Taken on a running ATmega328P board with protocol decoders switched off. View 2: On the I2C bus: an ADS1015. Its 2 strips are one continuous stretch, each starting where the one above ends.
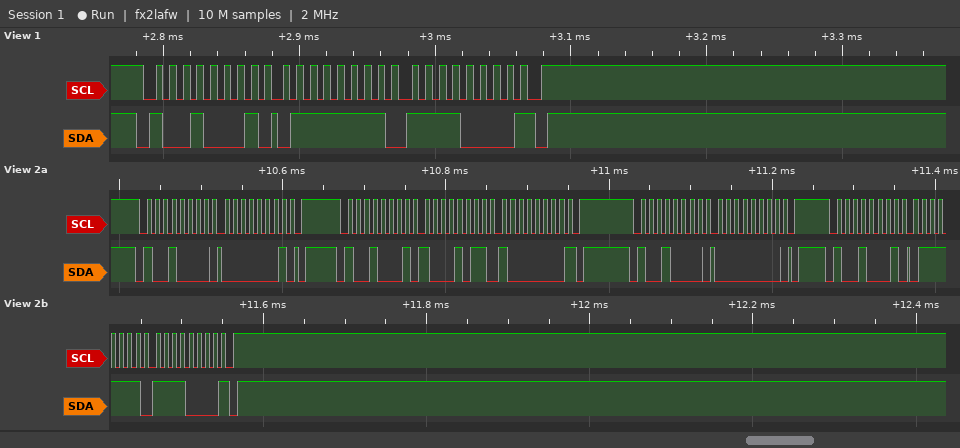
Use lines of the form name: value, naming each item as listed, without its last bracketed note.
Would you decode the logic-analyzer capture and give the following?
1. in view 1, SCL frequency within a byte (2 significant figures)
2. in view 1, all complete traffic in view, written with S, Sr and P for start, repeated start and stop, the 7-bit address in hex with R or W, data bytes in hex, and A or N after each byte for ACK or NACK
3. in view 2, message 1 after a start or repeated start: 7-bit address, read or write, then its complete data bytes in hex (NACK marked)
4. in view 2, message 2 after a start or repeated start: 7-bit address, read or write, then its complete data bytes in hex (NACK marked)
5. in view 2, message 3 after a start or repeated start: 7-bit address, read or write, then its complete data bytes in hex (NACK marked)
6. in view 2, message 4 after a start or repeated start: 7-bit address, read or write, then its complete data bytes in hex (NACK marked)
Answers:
in view 1, SCL frequency within a byte: 100 kHz
in view 1, all complete traffic in view, written with S, Sr and P for start, repeated start and stop, the 7-bit address in hex with R or W, data bytes in hex, and A or N after each byte for ACK or NACK: S 48R A 7F A F0 N P
in view 2, message 1 after a start or repeated start: 7-bit address, read or write, then its complete data bytes in hex: 0x48 write: 01
in view 2, message 2 after a start or repeated start: 7-bit address, read or write, then its complete data bytes in hex: 0x48 read: 8B 80 NACK
in view 2, message 3 after a start or repeated start: 7-bit address, read or write, then its complete data bytes in hex: 0x48 write: 00
in view 2, message 4 after a start or repeated start: 7-bit address, read or write, then its complete data bytes in hex: 0x48 read: 7F F0 NACK
